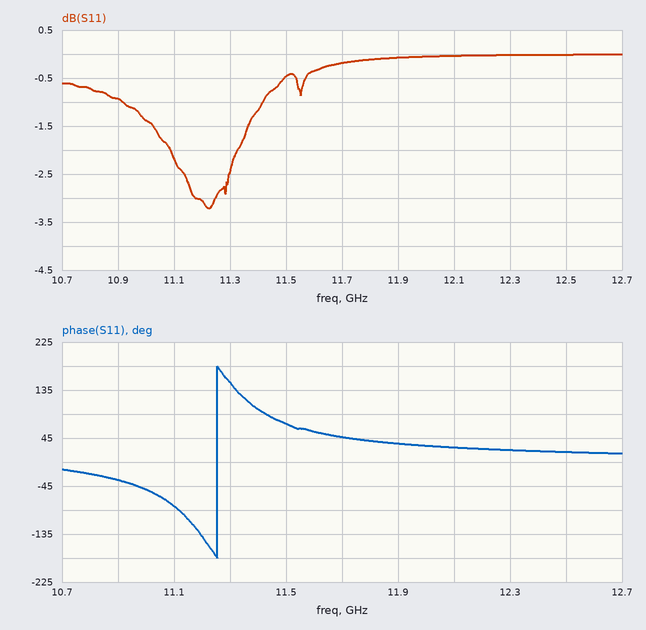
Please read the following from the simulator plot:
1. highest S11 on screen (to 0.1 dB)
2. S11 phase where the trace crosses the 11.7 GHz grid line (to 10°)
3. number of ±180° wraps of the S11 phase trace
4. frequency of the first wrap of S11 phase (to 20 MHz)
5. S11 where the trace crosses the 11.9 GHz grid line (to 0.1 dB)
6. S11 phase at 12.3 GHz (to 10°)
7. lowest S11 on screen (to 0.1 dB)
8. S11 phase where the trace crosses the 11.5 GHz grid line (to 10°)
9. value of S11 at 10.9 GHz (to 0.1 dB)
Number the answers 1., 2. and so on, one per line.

1. 0.0 dB
2. 50°
3. 1
4. 11.26 GHz
5. -0.1 dB
6. 20°
7. -3.2 dB
8. 70°
9. -0.9 dB
